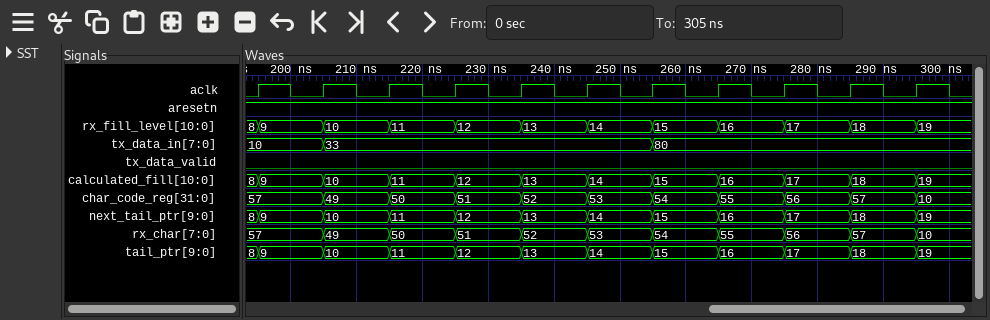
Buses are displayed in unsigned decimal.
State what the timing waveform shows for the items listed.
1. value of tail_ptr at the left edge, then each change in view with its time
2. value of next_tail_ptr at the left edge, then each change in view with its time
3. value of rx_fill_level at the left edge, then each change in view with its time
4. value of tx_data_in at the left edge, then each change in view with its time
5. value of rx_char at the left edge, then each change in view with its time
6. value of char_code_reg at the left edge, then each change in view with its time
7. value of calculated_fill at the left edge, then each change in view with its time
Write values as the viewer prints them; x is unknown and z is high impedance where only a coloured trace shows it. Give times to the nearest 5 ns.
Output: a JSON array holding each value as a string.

["8, 9 at 195 ns, 10 at 205 ns, 11 at 215 ns, 12 at 225 ns, 13 at 235 ns, 14 at 245 ns, 15 at 255 ns, 16 at 265 ns, 17 at 275 ns, 18 at 285 ns, 19 at 295 ns", "8, 9 at 195 ns, 10 at 205 ns, 11 at 215 ns, 12 at 225 ns, 13 at 235 ns, 14 at 245 ns, 15 at 255 ns, 16 at 265 ns, 17 at 275 ns, 18 at 285 ns, 19 at 295 ns", "8, 9 at 195 ns, 10 at 205 ns, 11 at 215 ns, 12 at 225 ns, 13 at 235 ns, 14 at 245 ns, 15 at 255 ns, 16 at 265 ns, 17 at 275 ns, 18 at 285 ns, 19 at 295 ns", "10, 33 at 205 ns, 80 at 255 ns", "57, 49 at 205 ns, 50 at 215 ns, 51 at 225 ns, 52 at 235 ns, 53 at 245 ns, 54 at 255 ns, 55 at 265 ns, 56 at 275 ns, 57 at 285 ns, 10 at 295 ns", "57, 49 at 205 ns, 50 at 215 ns, 51 at 225 ns, 52 at 235 ns, 53 at 245 ns, 54 at 255 ns, 55 at 265 ns, 56 at 275 ns, 57 at 285 ns, 10 at 295 ns", "8, 9 at 195 ns, 10 at 205 ns, 11 at 215 ns, 12 at 225 ns, 13 at 235 ns, 14 at 245 ns, 15 at 255 ns, 16 at 265 ns, 17 at 275 ns, 18 at 285 ns, 19 at 295 ns"]
